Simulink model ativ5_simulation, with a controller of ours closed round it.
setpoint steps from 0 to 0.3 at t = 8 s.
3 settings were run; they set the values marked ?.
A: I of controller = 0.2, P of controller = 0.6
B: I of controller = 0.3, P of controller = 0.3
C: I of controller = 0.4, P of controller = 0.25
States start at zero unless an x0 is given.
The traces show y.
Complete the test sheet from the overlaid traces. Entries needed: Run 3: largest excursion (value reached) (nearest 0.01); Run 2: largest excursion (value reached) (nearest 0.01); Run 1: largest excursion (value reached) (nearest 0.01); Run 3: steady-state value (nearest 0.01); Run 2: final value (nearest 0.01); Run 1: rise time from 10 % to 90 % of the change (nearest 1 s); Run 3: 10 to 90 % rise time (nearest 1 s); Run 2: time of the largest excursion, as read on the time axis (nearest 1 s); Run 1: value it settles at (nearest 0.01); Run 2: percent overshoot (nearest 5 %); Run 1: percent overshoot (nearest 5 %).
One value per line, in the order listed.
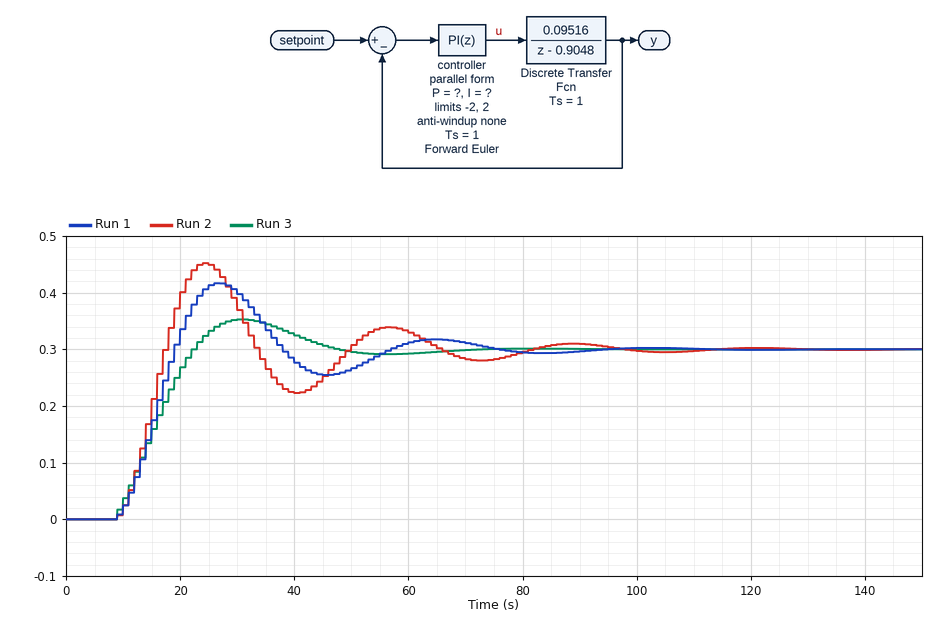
0.35
0.45
0.42
0.30
0.30
7 s
11 s
24 s
0.30
50 %
40 %
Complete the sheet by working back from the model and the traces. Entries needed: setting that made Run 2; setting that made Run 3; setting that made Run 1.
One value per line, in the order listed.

C
A
B
